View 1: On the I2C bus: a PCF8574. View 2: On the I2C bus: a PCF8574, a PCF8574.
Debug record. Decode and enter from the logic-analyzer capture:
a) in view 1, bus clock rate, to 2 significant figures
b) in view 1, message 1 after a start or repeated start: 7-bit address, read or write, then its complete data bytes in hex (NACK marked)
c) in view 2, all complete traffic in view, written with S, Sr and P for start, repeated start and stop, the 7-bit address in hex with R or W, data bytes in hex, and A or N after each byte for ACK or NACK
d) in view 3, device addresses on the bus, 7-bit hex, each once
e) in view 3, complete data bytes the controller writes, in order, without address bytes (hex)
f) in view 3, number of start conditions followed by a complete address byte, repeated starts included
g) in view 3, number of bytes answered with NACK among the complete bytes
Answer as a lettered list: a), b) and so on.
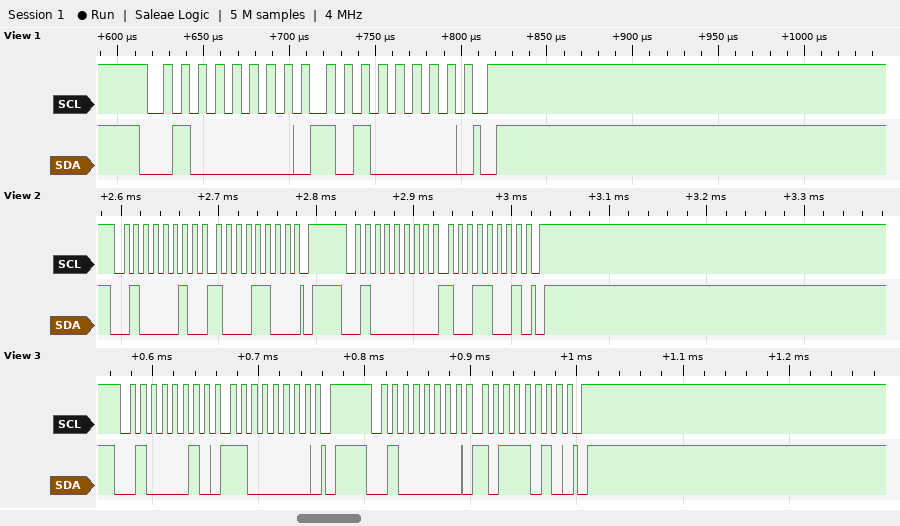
a) 100 kHz
b) 0x20 write: A0
c) S 21W A 8C A P S 20W A 99 A P
d) 0x21 0x20
e) C0 BA
f) 2
g) 0
